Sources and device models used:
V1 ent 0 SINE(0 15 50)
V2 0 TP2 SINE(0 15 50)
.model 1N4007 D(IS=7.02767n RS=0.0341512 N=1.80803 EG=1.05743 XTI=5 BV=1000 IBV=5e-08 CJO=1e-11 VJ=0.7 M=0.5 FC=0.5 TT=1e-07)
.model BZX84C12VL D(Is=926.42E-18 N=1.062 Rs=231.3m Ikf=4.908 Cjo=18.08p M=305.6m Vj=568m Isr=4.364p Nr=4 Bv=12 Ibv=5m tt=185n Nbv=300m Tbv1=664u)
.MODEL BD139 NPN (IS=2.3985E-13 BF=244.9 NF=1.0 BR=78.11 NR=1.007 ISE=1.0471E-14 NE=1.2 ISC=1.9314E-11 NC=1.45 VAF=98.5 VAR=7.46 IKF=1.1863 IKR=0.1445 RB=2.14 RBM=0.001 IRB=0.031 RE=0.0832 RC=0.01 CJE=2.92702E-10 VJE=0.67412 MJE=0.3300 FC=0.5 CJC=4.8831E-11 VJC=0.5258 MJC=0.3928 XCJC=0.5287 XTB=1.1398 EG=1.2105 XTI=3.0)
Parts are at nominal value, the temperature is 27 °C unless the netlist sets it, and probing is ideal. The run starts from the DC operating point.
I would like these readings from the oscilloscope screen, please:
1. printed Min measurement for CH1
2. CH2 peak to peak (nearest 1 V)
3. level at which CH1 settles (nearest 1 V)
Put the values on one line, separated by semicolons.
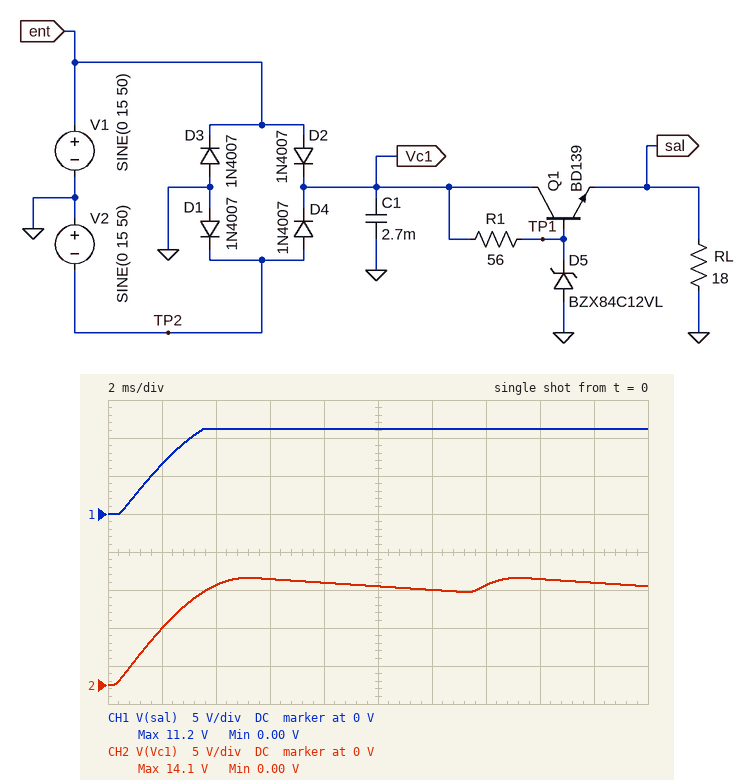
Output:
0.00 V; 14 V; 11 V
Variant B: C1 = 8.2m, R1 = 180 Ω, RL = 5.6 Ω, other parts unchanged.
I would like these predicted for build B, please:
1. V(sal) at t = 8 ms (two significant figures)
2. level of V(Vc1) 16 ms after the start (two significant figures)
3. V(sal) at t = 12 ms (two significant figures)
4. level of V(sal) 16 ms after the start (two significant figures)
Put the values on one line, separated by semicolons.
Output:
9.1 V; 14 V; 8.6 V; 9.4 V
